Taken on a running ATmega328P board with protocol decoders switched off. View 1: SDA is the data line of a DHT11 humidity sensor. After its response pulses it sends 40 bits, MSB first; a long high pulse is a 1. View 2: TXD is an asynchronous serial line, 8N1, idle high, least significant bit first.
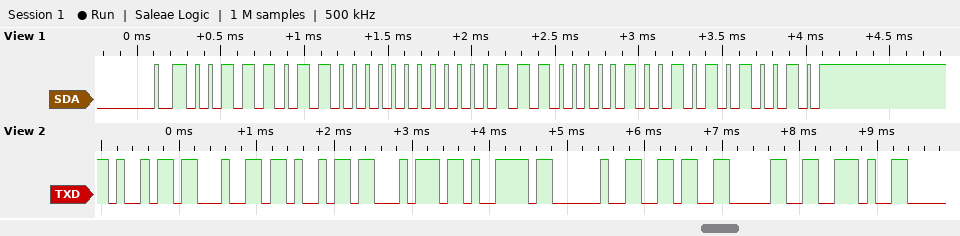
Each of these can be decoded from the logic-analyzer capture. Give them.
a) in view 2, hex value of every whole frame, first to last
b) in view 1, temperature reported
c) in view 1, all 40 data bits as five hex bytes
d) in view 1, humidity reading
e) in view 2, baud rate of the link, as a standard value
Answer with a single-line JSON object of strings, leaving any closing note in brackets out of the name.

{"in view 2, hex value of every whole frame, first to last": "0x69 0x64 0x69 0x74 0x79 0x20 0x36 0x30 0x2E", "in view 1, temperature reported": "14.9 °C", "in view 1, all 40 data bits as five hex bytes": "3B 00 0E 09 52", "in view 1, humidity reading": "59 %", "in view 2, baud rate of the link, as a standard value": "9600 baud"}
